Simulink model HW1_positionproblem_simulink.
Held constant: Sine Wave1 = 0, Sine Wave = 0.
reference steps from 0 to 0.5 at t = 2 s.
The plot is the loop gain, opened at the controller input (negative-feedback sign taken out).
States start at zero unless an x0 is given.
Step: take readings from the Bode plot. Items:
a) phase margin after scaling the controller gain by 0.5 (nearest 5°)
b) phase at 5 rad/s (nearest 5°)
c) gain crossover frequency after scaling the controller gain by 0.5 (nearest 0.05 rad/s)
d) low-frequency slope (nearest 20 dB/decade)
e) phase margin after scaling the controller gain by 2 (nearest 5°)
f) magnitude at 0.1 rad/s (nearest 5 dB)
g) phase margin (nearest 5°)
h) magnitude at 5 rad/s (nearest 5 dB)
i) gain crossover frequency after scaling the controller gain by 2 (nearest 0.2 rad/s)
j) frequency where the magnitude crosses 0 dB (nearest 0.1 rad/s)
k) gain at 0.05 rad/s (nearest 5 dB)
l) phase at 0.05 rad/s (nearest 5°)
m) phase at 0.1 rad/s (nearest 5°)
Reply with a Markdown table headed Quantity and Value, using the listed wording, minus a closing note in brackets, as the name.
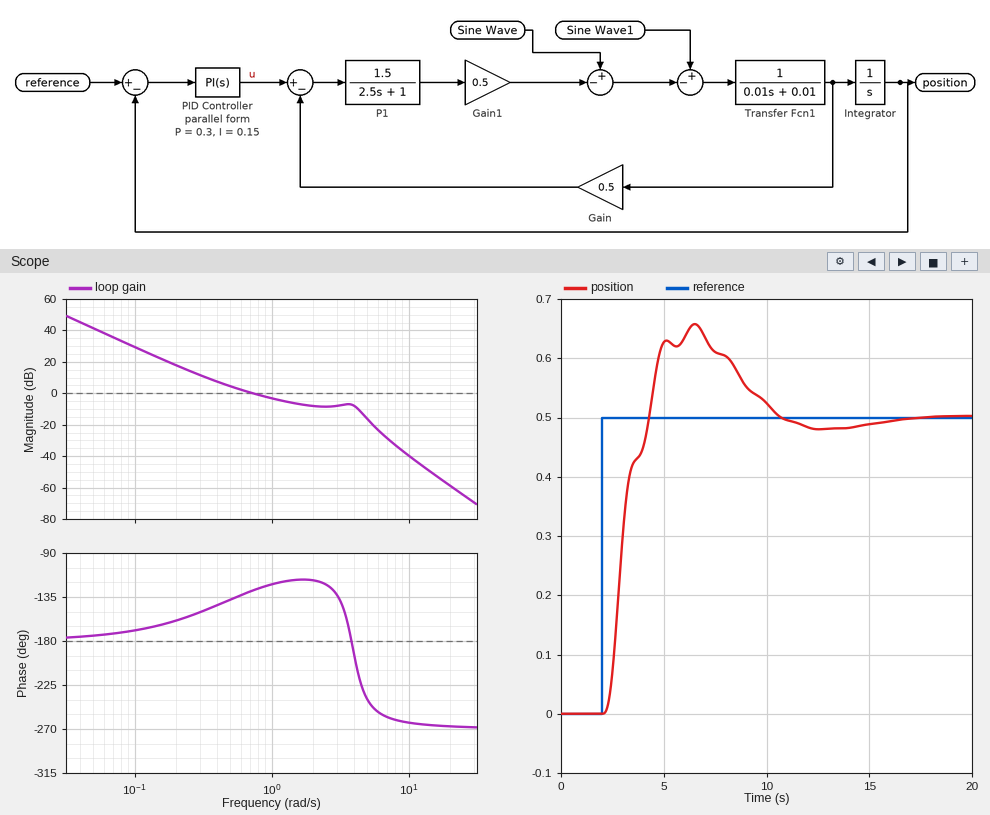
| Quantity | Value |
|---|---|
| phase margin after scaling the controller gain by 0.5 | 40° |
| phase at 5 rad/s | -240° |
| gain crossover frequency after scaling the controller gain by 0.5 | 0.45 rad/s |
| low-frequency slope | -40 dB/decade |
| phase margin after scaling the controller gain by 2 | 60° |
| magnitude at 0.1 rad/s | 30 dB |
| phase margin | 50° |
| magnitude at 5 rad/s | -15 dB |
| gain crossover frequency after scaling the controller gain by 2 | 1.4 rad/s |
| frequency where the magnitude crosses 0 dB | 0.7 rad/s |
| gain at 0.05 rad/s | 40 dB |
| phase at 0.05 rad/s | -175° |
| phase at 0.1 rad/s | -170° |
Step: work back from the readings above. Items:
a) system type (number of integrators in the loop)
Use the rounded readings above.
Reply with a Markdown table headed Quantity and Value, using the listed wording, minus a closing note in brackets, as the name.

| Quantity | Value |
|---|---|
| system type | 2 |
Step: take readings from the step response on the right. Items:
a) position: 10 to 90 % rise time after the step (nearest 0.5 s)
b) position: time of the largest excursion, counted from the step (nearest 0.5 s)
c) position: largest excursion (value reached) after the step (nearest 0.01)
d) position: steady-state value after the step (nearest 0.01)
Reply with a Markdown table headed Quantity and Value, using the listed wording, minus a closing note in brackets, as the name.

| Quantity | Value |
|---|---|
| position: 10 to 90 % rise time after the step | 1.5 s |
| position: time of the largest excursion, counted from the step | 4.5 s |
| position: largest excursion (value reached) after the step | 0.66 |
| position: steady-state value after the step | 0.50 |
